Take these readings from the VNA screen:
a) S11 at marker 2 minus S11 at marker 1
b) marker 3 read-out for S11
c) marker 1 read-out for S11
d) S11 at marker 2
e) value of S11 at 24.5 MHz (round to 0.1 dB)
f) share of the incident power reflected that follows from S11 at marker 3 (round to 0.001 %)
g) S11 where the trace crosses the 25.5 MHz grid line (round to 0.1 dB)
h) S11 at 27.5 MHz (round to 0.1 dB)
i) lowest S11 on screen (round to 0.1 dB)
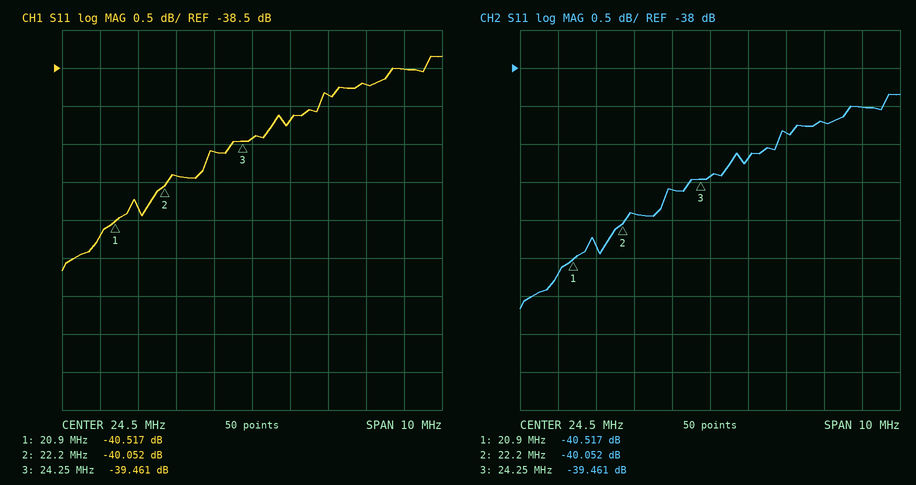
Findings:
0.465 dB
-39.461 dB
-40.517 dB
-40.052 dB
-39.4 dB
0.011 %
-39.2 dB
-38.7 dB
-41.2 dB
